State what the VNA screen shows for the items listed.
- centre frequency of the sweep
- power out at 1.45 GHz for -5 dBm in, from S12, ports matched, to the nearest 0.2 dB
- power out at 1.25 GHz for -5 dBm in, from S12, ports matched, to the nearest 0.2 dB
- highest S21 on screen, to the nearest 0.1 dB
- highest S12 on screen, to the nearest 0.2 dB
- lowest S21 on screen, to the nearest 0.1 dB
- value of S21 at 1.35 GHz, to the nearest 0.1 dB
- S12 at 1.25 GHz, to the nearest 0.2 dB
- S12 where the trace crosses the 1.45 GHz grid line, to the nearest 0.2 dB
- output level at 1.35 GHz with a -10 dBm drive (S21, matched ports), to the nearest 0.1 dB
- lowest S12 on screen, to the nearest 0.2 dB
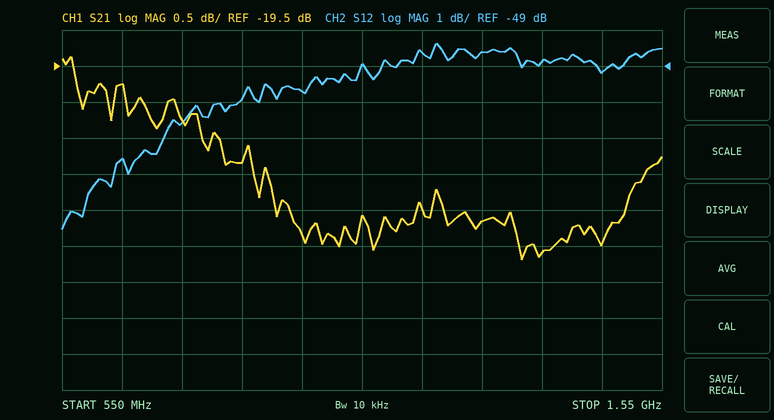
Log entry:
1.05 GHz
-54.2 dBm
-53.6 dBm
-19.4 dB
-48.4 dB
-22.2 dB
-22.1 dB
-48.6 dB
-49.2 dB
-32.1 dBm
-53.6 dB
